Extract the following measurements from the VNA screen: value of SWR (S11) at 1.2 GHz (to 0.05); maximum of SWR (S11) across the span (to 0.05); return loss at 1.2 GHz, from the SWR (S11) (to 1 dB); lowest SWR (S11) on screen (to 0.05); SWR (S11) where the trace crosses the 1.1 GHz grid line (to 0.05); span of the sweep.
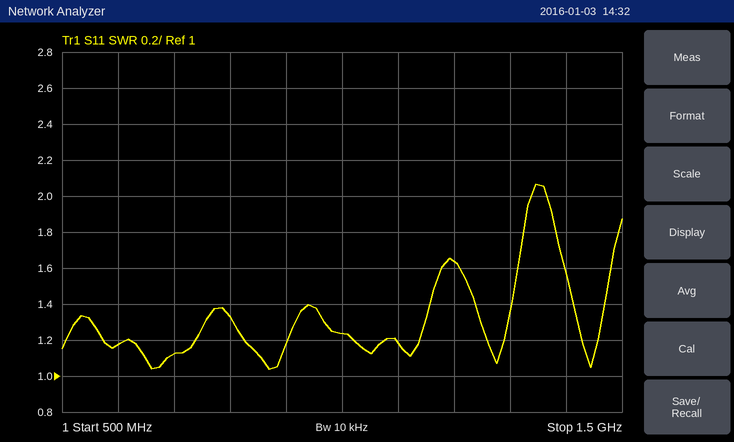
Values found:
1.65
2.05
12 dB
1.05
1.20
1 GHz
